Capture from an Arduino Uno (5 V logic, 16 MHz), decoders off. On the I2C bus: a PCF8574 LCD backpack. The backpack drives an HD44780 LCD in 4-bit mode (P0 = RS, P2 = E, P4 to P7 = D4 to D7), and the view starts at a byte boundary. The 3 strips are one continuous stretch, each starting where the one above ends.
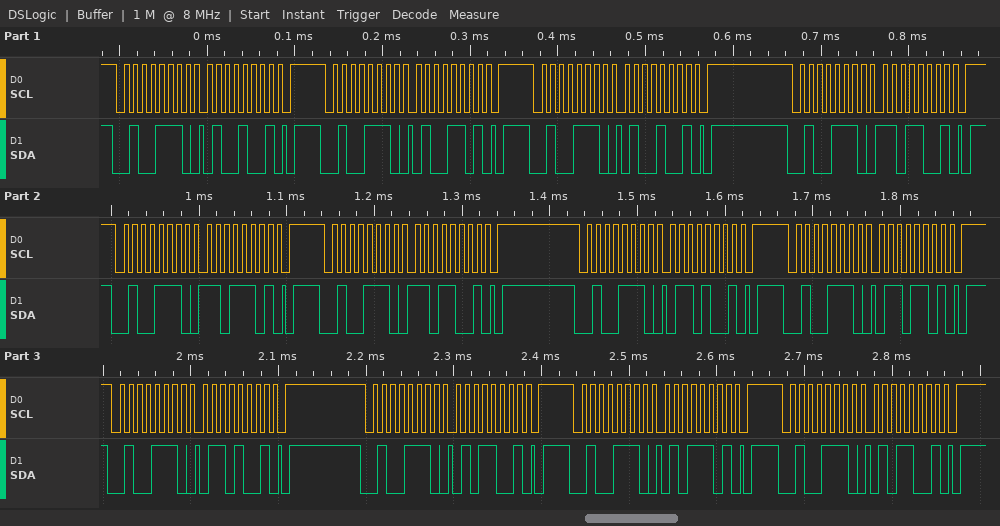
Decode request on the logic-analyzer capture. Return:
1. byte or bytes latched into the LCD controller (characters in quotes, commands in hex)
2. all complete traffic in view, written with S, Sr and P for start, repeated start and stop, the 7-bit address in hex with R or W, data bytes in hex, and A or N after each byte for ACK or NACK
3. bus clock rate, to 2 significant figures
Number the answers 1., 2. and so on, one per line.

1. 'M' 'e'
2. S 27W A 49 A P S 27W A 4D A P S 27W A 49 A P S 27W A D9 A P S 27W A DD A P S 27W A D9 A P S 27W A 69 A P S 27W A 6D A P S 27W A 69 A P S 27W A 59 A P S 27W A 5D A P S 27W A 59 A P
3. 100 kHz
